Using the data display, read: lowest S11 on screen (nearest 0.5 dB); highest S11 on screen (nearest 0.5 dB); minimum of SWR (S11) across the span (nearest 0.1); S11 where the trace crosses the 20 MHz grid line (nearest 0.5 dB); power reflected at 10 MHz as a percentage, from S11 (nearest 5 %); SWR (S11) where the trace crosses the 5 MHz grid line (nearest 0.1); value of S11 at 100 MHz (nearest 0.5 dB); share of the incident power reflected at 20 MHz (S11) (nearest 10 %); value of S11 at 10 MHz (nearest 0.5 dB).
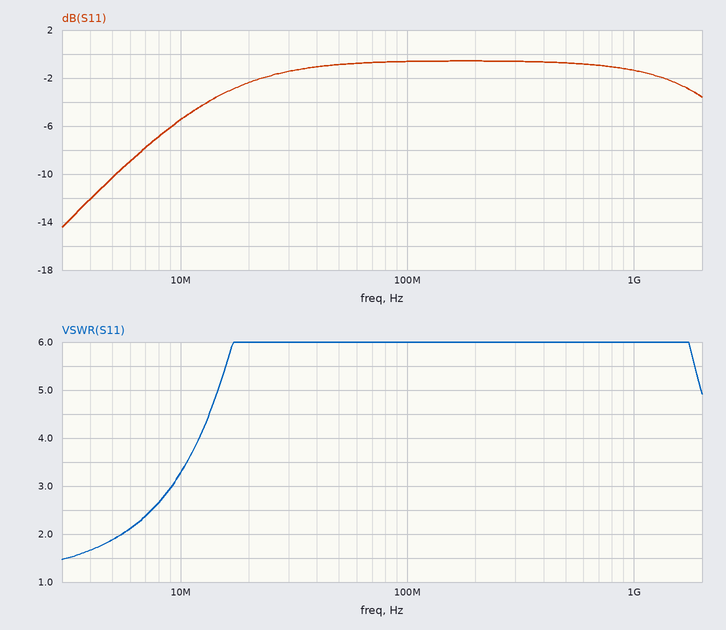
-14.5 dB
-0.5 dB
1.5
-2.5 dB
30 %
1.9
-0.5 dB
60 %
-5.5 dB
